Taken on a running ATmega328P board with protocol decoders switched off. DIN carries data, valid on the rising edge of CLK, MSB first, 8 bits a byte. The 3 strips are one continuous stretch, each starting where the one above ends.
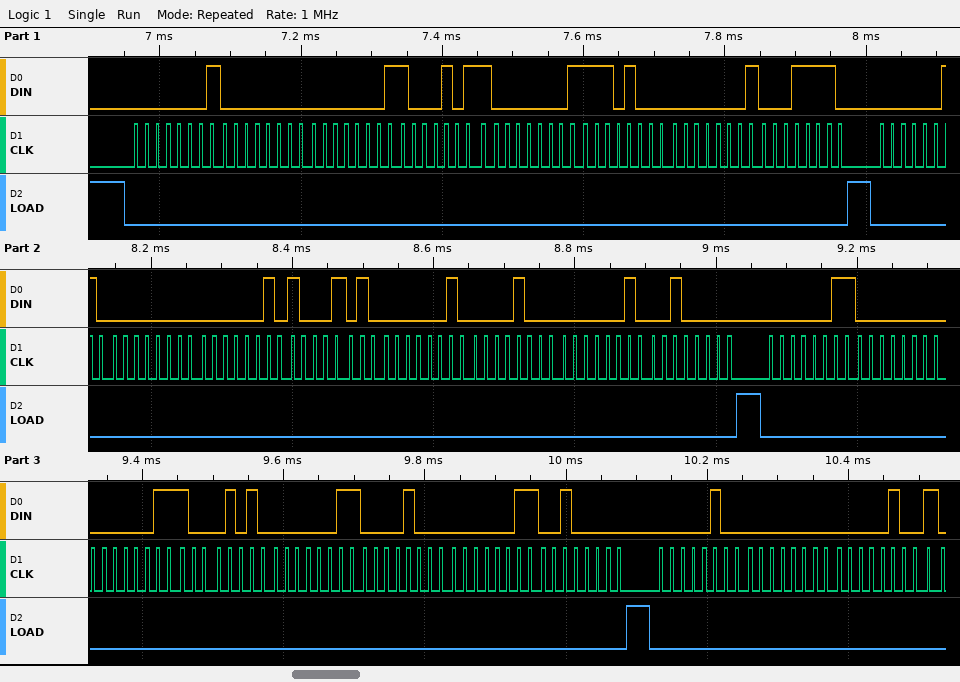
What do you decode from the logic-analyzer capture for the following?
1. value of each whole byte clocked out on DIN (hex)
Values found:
01 00 01 8B 01 E8 01 1E 02 00 02 8A 02 08 02 20 03 00 03 8A 03 08 03 20 04 00 04
